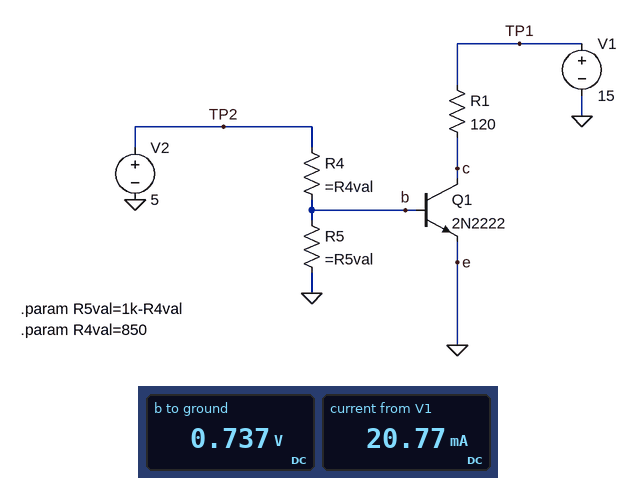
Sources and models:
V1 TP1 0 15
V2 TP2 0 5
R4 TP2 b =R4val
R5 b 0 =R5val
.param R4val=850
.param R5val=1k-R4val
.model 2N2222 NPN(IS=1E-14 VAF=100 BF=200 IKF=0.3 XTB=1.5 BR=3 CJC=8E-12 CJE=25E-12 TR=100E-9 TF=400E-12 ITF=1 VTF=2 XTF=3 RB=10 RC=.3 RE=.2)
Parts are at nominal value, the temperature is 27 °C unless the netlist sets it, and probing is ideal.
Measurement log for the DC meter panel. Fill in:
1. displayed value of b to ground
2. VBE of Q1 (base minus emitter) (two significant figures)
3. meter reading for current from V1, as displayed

0.737 V
740 mV
20.77 mA
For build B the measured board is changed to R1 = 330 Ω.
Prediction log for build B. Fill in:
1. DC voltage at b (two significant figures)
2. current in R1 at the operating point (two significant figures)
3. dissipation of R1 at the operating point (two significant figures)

740 mV
20 mA
130 mW
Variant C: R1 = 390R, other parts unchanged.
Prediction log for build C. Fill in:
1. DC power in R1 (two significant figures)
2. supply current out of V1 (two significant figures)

150 mW
20 mA
